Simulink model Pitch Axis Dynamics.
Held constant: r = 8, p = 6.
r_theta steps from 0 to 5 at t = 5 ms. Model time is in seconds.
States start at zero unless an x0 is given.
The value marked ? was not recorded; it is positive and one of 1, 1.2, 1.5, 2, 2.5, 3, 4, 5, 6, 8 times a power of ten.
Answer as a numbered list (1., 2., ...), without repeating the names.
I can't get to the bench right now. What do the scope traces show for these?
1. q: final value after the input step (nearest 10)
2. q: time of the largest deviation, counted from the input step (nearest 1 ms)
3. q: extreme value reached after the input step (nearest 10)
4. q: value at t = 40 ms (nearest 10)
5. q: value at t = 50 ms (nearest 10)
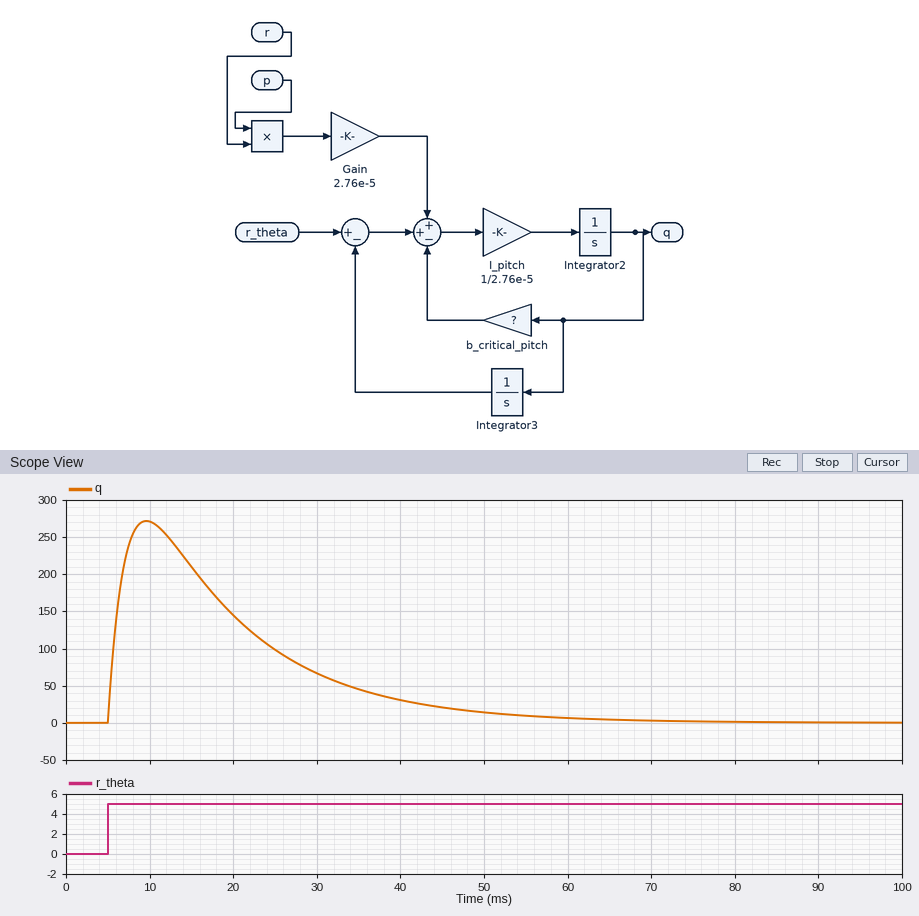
1. 0
2. 5 ms
3. 270
4. 30
5. 10
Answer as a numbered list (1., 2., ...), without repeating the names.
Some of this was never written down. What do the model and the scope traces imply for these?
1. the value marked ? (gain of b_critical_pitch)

1. 0.015
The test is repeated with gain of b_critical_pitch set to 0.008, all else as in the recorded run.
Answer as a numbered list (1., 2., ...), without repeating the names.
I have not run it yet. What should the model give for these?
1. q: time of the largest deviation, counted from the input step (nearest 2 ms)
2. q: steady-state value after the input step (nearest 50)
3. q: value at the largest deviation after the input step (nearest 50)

1. 6 ms
2. 0
3. 400
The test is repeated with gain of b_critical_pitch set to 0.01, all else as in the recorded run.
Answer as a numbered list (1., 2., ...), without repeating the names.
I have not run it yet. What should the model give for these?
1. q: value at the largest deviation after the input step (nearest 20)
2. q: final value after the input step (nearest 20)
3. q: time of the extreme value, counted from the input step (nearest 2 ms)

1. 360
2. 0
3. 6 ms
